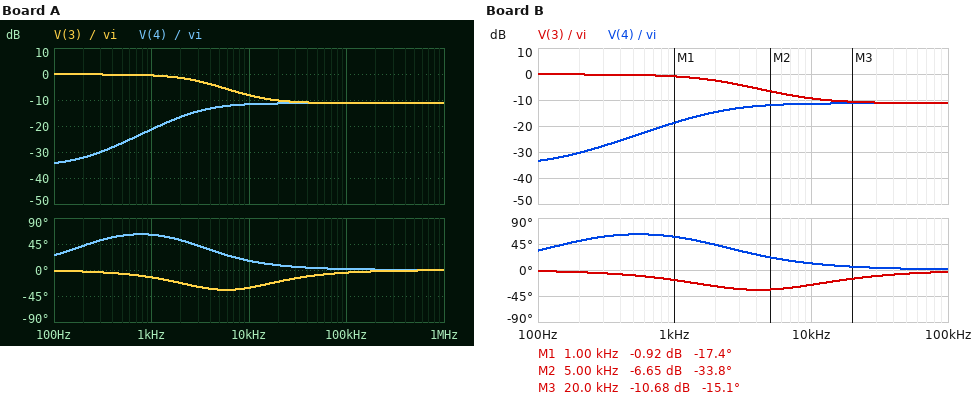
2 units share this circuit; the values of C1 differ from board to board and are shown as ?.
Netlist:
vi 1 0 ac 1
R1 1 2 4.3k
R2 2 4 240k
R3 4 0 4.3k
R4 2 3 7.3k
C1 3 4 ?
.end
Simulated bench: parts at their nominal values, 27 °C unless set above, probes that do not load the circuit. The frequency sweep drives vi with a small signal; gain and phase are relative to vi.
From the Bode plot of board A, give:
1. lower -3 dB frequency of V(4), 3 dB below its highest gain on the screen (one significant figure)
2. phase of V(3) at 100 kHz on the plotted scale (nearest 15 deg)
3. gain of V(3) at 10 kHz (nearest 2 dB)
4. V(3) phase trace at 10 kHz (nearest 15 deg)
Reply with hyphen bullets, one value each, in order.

- 3 kHz
- 0 deg
- -8 dB
- -30 deg
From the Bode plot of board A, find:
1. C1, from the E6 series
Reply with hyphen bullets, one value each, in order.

- 3.3 nF
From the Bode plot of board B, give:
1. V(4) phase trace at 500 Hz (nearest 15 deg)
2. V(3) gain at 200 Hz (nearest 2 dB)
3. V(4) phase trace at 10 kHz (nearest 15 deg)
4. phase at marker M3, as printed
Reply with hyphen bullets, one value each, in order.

- 60 deg
- 0 dB
- 15 deg
- -15.1 deg
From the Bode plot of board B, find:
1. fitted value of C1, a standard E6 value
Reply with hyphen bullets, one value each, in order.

- 4.7 nF
